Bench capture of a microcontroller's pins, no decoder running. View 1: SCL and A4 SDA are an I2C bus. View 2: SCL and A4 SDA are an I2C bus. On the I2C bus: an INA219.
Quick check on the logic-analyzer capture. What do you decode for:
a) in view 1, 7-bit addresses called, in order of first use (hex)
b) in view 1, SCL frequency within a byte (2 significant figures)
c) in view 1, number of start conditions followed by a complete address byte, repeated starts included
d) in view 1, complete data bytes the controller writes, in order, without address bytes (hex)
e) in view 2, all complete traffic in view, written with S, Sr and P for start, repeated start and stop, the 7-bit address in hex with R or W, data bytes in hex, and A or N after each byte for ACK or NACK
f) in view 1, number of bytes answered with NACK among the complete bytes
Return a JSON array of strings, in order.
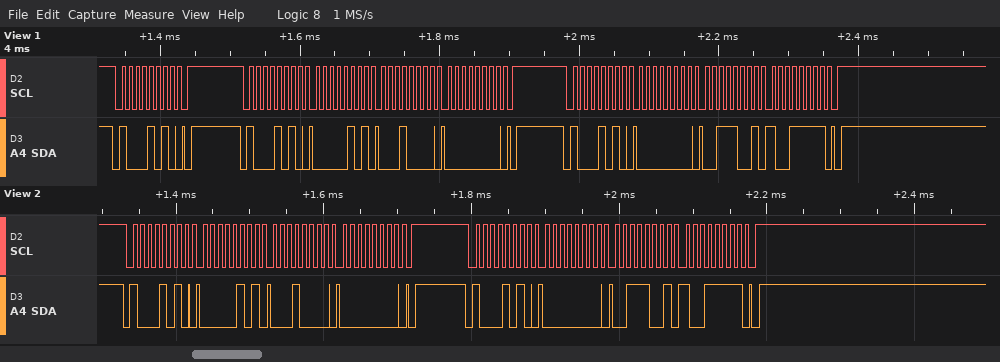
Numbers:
["0x45", "100 kHz", "3", "05 10 00 00 39 9F", "S 45W A 05 A 10 A 00 A P S 45W A 00 A 39 A 9F A P", "0"]
